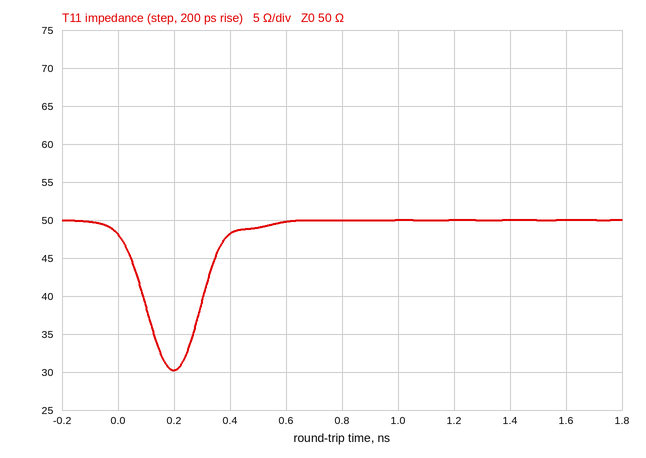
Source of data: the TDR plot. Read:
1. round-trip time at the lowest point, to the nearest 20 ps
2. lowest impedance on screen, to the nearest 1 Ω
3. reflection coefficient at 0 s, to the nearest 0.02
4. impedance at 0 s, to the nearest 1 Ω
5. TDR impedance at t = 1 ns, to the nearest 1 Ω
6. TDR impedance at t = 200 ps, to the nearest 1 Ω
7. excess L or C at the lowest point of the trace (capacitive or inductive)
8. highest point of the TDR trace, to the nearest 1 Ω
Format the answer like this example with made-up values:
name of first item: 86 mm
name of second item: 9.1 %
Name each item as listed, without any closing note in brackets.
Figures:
round-trip time at the lowest point, to the nearest 20 ps: 200 ps
lowest impedance on screen, to the nearest 1 Ω: 30 Ω
reflection coefficient at 0 s, to the nearest 0.02: -0.02
impedance at 0 s, to the nearest 1 Ω: 48 Ω
TDR impedance at t = 1 ns, to the nearest 1 Ω: 50 Ω
TDR impedance at t = 200 ps, to the nearest 1 Ω: 30 Ω
excess L or C at the lowest point of the trace: capacitive
highest point of the TDR trace, to the nearest 1 Ω: 50 Ω
